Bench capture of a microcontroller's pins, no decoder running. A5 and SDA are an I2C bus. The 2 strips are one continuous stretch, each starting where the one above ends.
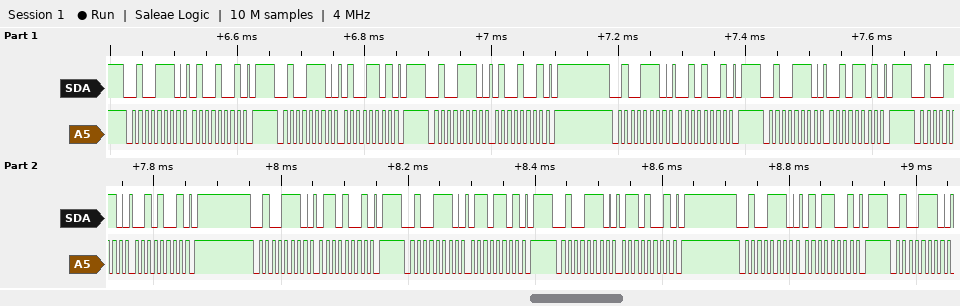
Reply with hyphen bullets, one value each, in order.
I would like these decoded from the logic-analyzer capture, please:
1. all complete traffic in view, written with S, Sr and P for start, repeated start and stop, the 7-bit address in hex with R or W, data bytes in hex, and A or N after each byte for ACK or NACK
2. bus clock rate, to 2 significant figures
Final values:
- S 27W A 49 A P S 27W A 4D A P S 27W A 49 A P S 27W A 29 A P S 27W A 2D A P S 27W A 29 A P S 27W A 69 A P S 27W A 6D A P S 27W A 69 A P S 27W A 59 A P S 27W A
- 100 kHz
